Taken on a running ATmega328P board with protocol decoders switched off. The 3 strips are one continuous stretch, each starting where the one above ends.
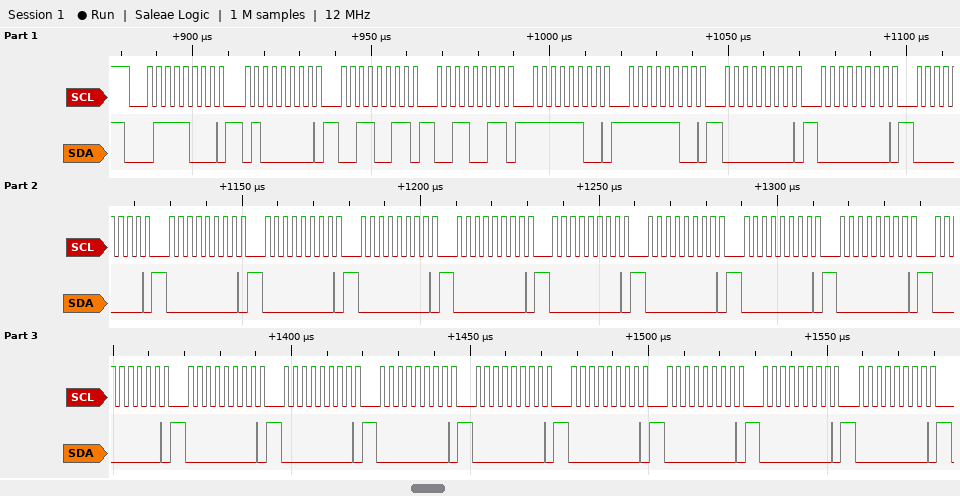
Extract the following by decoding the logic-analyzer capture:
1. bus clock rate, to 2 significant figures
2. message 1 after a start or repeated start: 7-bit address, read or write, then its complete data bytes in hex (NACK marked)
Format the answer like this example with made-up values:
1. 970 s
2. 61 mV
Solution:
1. 400 kHz
2. 0x3C write: 40 33 33 FC FC 00 00 00 00 00 00 00 00 00 00 00 00 00 00 00 00 00 00 00 00
